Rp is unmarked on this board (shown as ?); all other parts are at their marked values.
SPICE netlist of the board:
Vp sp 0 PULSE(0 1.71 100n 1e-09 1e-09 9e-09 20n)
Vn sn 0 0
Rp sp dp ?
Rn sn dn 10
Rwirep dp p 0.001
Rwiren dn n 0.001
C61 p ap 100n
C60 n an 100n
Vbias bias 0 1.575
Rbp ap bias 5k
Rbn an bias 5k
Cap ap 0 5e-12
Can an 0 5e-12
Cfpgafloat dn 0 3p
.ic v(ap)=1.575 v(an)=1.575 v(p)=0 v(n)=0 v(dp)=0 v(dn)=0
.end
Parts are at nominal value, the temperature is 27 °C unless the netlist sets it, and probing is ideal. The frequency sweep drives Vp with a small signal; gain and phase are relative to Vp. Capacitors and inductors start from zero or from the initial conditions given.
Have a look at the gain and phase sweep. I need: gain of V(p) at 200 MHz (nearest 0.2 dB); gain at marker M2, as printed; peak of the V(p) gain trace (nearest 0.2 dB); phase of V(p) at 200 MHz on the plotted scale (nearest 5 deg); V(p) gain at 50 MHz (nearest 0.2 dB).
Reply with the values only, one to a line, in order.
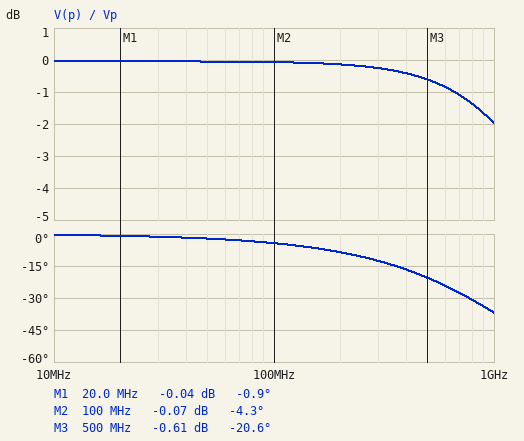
-0.2 dB
-0.07 dB
0 dB
-10 deg
0 dB
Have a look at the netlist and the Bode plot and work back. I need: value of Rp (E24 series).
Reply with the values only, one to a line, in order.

24 Ω
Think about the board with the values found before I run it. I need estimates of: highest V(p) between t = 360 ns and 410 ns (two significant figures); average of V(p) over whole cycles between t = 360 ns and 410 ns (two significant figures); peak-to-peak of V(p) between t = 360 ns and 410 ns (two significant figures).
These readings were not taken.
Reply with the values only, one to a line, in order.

1.7 V
850 mV
1.7 V
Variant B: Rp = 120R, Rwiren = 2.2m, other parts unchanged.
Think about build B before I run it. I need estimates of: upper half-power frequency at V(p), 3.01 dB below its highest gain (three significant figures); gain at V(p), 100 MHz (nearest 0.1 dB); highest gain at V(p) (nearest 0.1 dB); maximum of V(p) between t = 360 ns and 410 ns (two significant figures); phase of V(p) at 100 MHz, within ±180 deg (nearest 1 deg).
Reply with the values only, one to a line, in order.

272 MHz
-0.8 dB
-0.2 dB
1.7 V
-20 deg
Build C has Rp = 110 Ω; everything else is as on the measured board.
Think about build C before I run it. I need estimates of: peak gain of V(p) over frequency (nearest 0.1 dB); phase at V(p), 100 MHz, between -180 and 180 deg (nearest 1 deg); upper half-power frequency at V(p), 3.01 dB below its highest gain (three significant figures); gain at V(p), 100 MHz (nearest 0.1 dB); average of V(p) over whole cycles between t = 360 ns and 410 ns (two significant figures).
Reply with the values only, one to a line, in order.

-0.2 dB
-19 deg
296 MHz
-0.7 dB
840 mV
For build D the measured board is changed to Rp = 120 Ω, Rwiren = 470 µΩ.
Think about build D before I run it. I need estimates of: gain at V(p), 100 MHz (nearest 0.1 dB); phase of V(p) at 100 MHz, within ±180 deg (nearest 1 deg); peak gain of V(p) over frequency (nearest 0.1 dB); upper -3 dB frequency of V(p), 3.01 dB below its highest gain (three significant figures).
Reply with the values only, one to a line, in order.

-0.8 dB
-20 deg
-0.2 dB
272 MHz
